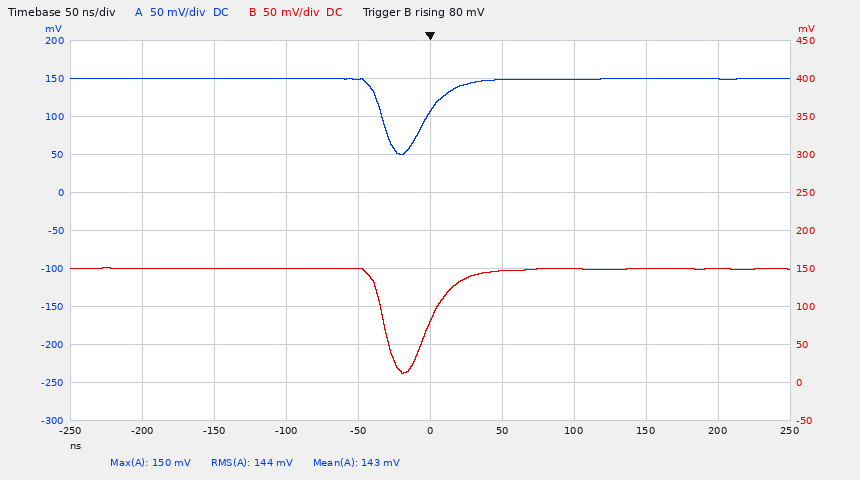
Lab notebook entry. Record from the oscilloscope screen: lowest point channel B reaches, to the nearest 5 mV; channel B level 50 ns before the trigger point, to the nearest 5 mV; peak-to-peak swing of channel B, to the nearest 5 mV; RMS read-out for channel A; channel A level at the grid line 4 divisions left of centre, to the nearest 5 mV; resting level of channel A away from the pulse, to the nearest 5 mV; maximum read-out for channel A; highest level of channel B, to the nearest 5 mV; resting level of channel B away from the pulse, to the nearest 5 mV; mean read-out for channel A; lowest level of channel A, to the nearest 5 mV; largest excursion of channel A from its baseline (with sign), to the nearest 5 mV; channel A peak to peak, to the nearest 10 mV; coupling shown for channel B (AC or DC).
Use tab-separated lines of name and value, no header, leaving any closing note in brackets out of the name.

lowest point channel B reaches, to the nearest 5 mV	10 mV
channel B level 50 ns before the trigger point, to the nearest 5 mV	150 mV
peak-to-peak swing of channel B, to the nearest 5 mV	140 mV
RMS read-out for channel A	144 mV
channel A level at the grid line 4 divisions left of centre, to the nearest 5 mV	150 mV
resting level of channel A away from the pulse, to the nearest 5 mV	150 mV
maximum read-out for channel A	150 mV
highest level of channel B, to the nearest 5 mV	150 mV
resting level of channel B away from the pulse, to the nearest 5 mV	150 mV
mean read-out for channel A	143 mV
lowest level of channel A, to the nearest 5 mV	50 mV
largest excursion of channel A from its baseline (with sign), to the nearest 5 mV	-100 mV
channel A peak to peak, to the nearest 10 mV	100 mV
coupling shown for channel B	DC
